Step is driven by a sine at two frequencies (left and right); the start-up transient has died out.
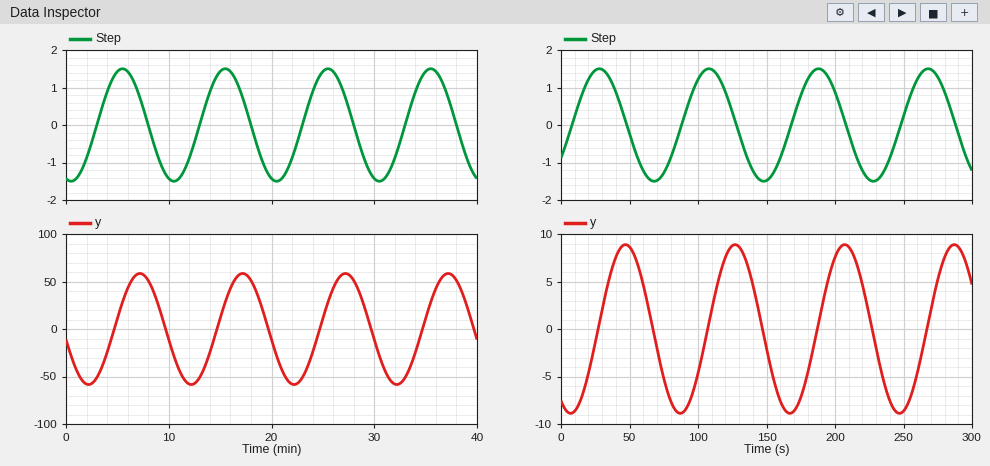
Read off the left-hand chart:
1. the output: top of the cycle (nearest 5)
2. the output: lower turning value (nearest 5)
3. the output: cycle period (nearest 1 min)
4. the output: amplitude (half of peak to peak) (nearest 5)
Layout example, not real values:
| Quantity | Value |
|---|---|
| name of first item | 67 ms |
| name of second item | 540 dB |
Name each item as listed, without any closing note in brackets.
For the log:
| Quantity | Value |
|---|---|
| the output: top of the cycle | 60 |
| the output: lower turning value | -60 |
| the output: cycle period | 10 min |
| the output: amplitude (half of peak to peak) | 60 |
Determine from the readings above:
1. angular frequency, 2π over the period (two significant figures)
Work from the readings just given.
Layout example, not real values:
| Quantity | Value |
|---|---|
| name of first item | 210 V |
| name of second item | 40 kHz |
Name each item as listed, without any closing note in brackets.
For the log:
| Quantity | Value |
|---|---|
| angular frequency, 2π over the period | 0.63 rad/min |
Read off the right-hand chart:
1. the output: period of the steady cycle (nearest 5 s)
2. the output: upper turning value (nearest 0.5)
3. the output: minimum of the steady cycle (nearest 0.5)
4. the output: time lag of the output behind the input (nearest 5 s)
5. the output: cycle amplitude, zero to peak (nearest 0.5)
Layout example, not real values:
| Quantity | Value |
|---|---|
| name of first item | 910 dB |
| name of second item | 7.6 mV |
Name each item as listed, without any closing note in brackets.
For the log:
| Quantity | Value |
|---|---|
| the output: period of the steady cycle | 80 s |
| the output: upper turning value | 9.0 |
| the output: minimum of the steady cycle | -9.0 |
| the output: time lag of the output behind the input | 20 s |
| the output: cycle amplitude, zero to peak | 9.0 |
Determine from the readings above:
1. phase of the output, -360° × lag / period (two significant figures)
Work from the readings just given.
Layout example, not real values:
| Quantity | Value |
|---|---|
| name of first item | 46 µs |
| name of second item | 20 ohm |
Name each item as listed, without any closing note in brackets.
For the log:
| Quantity | Value |
|---|---|
| phase of the output, -360° × lag / period | -90° |
